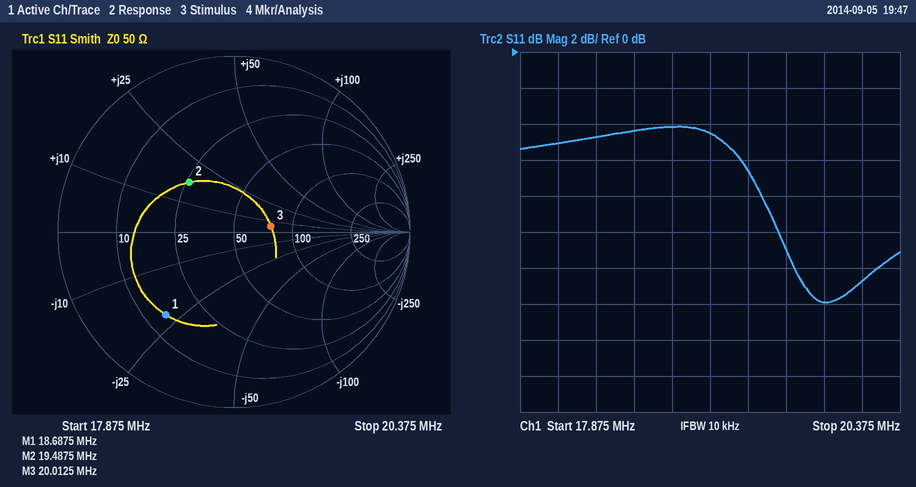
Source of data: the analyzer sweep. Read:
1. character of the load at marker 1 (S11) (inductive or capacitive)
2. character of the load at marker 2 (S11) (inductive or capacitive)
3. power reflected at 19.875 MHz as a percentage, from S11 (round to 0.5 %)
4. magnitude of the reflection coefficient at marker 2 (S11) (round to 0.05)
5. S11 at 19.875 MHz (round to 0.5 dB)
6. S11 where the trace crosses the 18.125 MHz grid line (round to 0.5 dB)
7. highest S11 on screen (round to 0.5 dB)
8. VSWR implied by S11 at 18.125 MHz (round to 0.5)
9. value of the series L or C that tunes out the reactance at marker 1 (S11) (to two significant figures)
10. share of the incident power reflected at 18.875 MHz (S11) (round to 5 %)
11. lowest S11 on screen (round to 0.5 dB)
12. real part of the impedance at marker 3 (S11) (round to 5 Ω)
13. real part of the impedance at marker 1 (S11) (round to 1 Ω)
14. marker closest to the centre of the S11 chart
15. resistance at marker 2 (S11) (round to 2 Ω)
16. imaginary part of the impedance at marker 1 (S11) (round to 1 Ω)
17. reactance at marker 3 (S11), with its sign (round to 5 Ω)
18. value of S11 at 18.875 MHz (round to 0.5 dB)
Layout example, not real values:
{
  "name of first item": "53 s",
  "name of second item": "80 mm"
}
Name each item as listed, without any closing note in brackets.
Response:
{
  "character of the load at marker 1 (S11)": "capacitive",
  "character of the load at marker 2 (S11)": "inductive",
  "power reflected at 19.875 MHz as a percentage, from S11": "4.0 %",
  "magnitude of the reflection coefficient at marker 2 (S11)": "0.40",
  "S11 at 19.875 MHz": "-14.0 dB",
  "S11 where the trace crosses the 18.125 MHz grid line": "-5.0 dB",
  "highest S11 on screen": "-4.0 dB",
  "VSWR implied by S11 at 18.125 MHz": "3.5",
  "value of the series L or C that tunes out the reactance at marker 1 (S11)": "190 nH",
  "share of the incident power reflected at 18.875 MHz (S11)": "40 %",
  "lowest S11 on screen": "-14.0 dB",
  "real part of the impedance at marker 3 (S11)": "75 Ω",
  "real part of the impedance at marker 1 (S11)": "15 Ω",
  "marker closest to the centre of the S11 chart": "marker 3",
  "resistance at marker 2 (S11)": "26 Ω",
  "imaginary part of the impedance at marker 1 (S11)": "-22 Ω",
  "reactance at marker 3 (S11), with its sign": "+5 Ω",
  "value of S11 at 18.875 MHz": "-4.0 dB"
}
